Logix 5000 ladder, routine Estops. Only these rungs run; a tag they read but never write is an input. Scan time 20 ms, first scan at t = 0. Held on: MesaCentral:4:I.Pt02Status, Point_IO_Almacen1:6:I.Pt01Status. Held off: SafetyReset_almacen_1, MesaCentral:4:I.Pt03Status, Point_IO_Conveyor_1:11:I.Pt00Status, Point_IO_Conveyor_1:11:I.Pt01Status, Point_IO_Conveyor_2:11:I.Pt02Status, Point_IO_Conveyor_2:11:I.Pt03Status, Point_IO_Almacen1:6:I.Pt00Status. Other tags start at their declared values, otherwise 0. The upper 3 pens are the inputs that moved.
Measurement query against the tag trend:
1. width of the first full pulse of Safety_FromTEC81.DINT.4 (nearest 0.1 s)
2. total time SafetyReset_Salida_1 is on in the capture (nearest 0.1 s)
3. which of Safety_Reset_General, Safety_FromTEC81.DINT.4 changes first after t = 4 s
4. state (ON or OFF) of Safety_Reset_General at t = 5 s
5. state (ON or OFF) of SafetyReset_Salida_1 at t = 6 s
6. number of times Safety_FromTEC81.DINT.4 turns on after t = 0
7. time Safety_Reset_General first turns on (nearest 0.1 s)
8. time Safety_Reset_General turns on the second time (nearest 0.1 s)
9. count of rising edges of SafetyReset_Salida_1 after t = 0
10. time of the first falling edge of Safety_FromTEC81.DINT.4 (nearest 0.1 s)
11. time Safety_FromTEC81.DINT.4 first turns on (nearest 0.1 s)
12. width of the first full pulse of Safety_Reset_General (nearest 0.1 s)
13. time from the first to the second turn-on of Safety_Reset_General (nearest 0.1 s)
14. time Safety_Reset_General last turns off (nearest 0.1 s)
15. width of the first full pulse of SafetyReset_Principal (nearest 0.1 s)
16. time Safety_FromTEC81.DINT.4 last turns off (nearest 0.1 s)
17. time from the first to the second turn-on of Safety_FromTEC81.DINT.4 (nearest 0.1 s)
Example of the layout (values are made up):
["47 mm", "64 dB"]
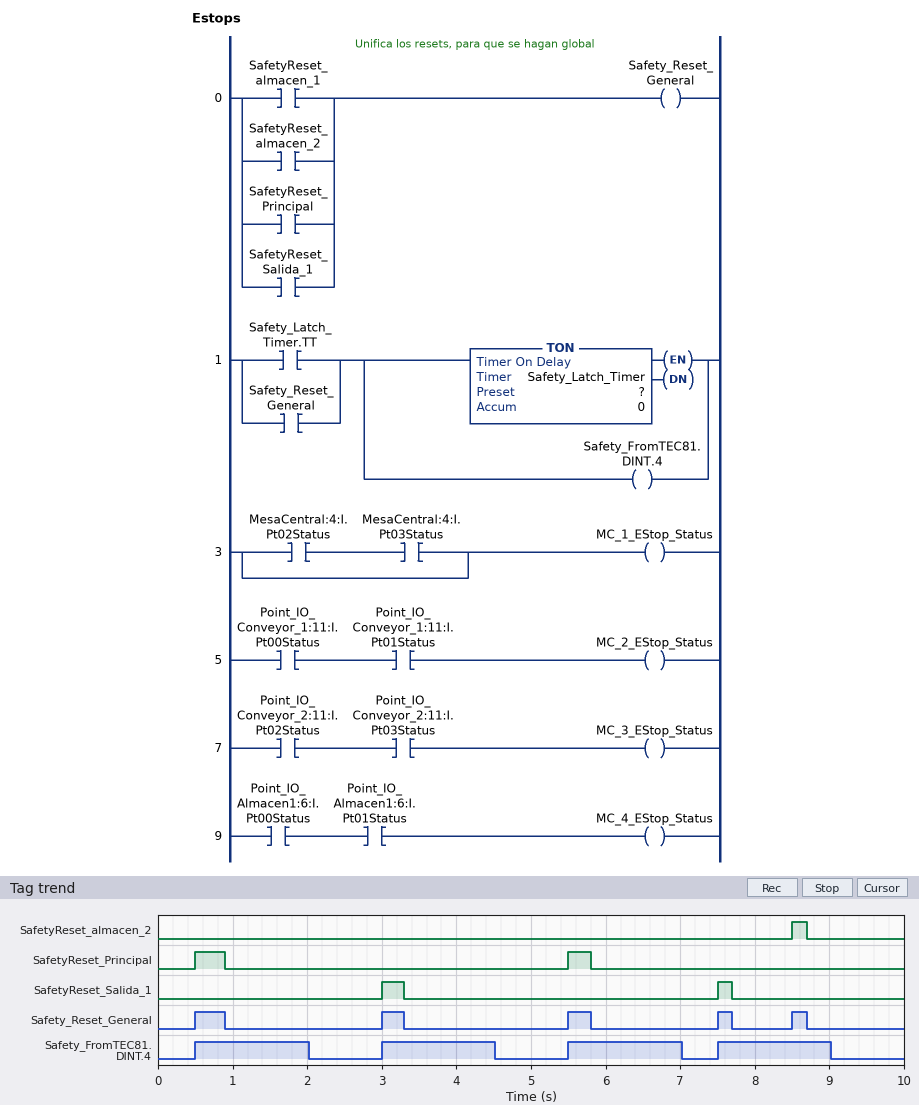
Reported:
["1.5 s", "0.5 s", "Safety_FromTEC81.DINT.4", "OFF", "OFF", "4", "0.5 s", "3.0 s", "2", "2.0 s", "0.5 s", "0.4 s", "2.5 s", "8.7 s", "0.4 s", "9.0 s", "2.5 s"]
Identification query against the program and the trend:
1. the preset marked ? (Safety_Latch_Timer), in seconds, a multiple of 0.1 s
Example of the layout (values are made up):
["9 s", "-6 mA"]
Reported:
["1.5 s"]
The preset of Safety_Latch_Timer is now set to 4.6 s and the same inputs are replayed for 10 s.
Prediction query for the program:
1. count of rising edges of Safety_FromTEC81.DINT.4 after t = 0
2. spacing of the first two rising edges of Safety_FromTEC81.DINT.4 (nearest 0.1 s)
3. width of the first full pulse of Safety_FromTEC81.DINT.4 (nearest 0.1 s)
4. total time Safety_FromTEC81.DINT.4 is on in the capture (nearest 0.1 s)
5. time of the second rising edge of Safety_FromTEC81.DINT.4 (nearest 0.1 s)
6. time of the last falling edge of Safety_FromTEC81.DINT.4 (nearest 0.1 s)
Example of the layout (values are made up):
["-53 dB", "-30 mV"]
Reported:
["2", "5.0 s", "4.6 s", "9.1 s", "5.5 s", "5.1 s"]
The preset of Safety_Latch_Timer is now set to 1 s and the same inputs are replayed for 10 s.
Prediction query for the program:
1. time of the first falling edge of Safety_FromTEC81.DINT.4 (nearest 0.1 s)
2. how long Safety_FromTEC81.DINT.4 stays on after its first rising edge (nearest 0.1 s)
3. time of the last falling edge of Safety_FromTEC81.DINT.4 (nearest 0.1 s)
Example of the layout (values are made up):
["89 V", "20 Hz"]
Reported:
["1.5 s", "1.0 s", "8.7 s"]
